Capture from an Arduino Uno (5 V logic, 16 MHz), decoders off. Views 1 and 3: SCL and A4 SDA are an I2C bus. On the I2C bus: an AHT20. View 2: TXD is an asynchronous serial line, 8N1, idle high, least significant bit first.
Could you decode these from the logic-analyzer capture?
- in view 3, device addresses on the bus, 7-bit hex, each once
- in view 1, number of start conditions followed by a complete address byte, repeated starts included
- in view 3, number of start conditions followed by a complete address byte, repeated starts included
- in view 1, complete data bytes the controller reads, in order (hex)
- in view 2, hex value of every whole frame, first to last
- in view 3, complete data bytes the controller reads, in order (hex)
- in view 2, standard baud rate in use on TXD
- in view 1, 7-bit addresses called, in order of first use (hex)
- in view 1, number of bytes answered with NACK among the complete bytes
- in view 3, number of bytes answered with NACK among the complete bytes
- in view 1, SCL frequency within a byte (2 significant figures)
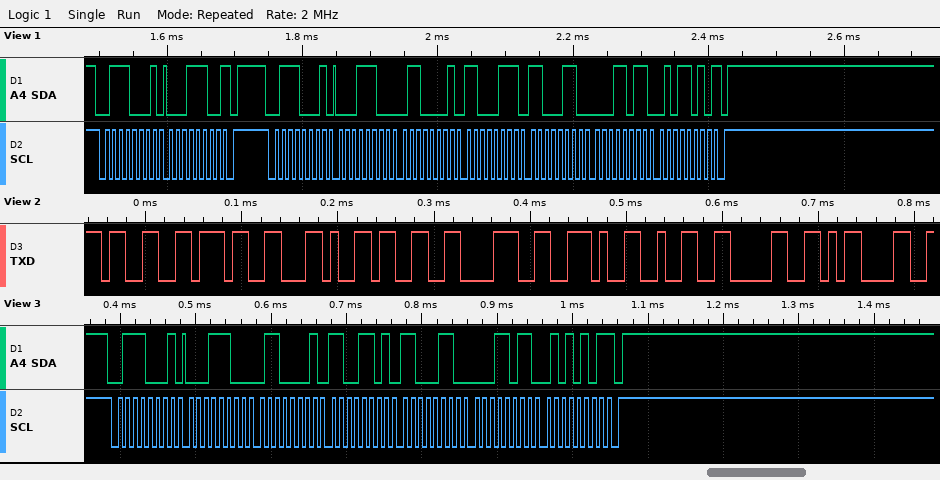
0x38
2
1
1C 1C 61 C7 C6 1B 5A
33 37 2C 33 38 2E 32 30 0D
1C 61 CD C6 1B 55
115200 baud
0x38
2
1
100 kHz
